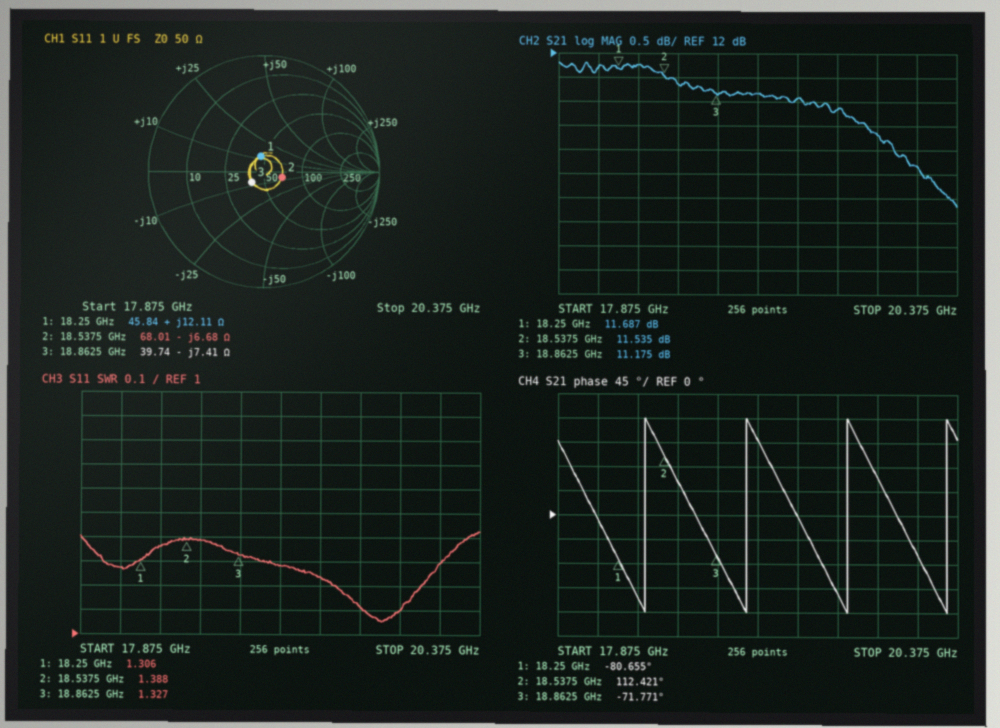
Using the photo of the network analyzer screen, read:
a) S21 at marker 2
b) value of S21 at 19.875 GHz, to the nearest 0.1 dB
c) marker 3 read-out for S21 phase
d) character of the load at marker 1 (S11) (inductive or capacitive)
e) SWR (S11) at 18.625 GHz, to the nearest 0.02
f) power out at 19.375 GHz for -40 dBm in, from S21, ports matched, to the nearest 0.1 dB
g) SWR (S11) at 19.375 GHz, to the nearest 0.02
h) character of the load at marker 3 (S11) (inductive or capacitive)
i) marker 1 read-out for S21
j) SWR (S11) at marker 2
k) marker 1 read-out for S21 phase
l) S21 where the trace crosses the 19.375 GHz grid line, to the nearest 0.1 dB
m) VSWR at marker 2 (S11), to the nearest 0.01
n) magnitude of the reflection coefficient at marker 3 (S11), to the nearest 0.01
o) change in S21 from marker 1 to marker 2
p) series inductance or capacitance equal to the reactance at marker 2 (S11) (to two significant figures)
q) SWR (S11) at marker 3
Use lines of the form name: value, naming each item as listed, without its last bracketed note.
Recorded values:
S21 at marker 2: 11.535 dB
value of S21 at 19.875 GHz, to the nearest 0.1 dB: 10.3 dB
marker 3 read-out for S21 phase: -71.771°
character of the load at marker 1 (S11): inductive
SWR (S11) at 18.625 GHz, to the nearest 0.02: 1.38
power out at 19.375 GHz for -40 dBm in, from S21, ports matched, to the nearest 0.1 dB: -28.9 dBm
SWR (S11) at 19.375 GHz, to the nearest 0.02: 1.24
character of the load at marker 3 (S11): capacitive
marker 1 read-out for S21: 11.687 dB
SWR (S11) at marker 2: 1.388
marker 1 read-out for S21 phase: -80.655°
S21 where the trace crosses the 19.375 GHz grid line, to the nearest 0.1 dB: 11.1 dB
VSWR at marker 2 (S11), to the nearest 0.01: 1.39
magnitude of the reflection coefficient at marker 3 (S11), to the nearest 0.01: 0.14
change in S21 from marker 1 to marker 2: -0.152 dB
series inductance or capacitance equal to the reactance at marker 2 (S11): 1.3 pF
SWR (S11) at marker 3: 1.327
